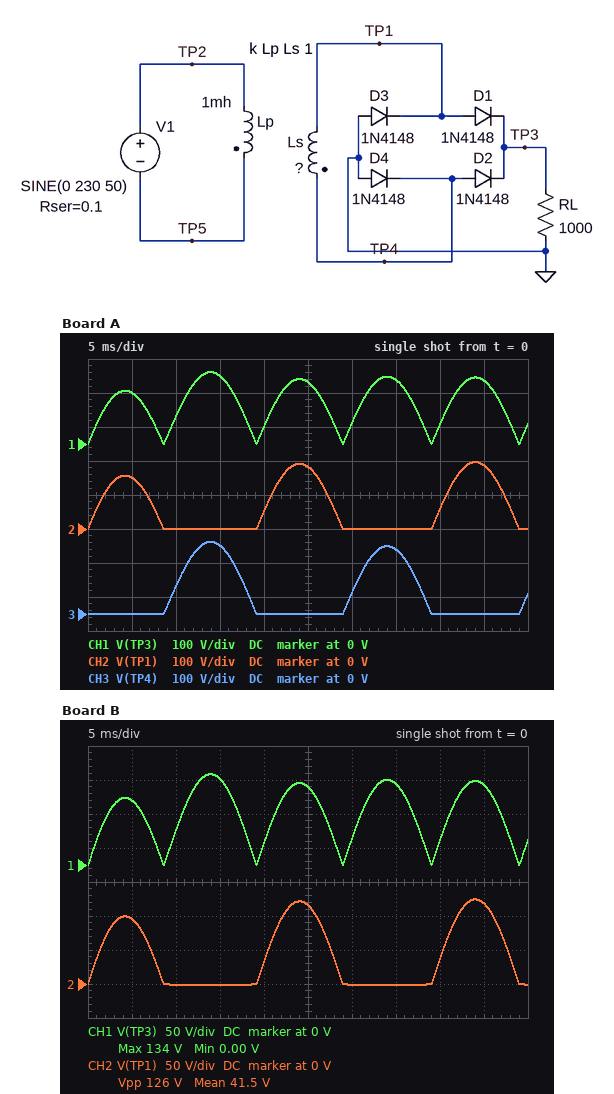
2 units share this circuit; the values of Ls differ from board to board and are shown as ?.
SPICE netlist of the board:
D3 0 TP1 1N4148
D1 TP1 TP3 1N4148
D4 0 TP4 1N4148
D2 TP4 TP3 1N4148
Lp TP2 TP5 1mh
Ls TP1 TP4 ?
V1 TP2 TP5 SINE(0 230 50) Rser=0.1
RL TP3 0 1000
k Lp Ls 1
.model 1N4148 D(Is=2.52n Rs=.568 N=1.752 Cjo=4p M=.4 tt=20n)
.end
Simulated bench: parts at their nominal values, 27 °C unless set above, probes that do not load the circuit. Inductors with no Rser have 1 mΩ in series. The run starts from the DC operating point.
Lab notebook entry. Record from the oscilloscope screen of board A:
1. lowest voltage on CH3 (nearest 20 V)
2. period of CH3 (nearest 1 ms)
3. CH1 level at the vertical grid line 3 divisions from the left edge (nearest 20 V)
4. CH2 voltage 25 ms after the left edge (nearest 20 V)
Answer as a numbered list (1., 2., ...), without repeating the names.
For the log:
1. 0 V
2. 20 ms
3. 200 V
4. 180 V
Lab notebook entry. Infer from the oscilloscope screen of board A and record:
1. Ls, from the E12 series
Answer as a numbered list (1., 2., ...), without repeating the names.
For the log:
1. 820 µH
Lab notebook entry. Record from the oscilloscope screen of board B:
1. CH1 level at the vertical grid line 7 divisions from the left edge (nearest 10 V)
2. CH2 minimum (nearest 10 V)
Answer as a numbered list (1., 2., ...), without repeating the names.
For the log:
1. 120 V
2. 0 V
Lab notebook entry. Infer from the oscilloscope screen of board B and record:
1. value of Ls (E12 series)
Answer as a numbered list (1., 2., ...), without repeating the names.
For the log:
1. 330 µH
